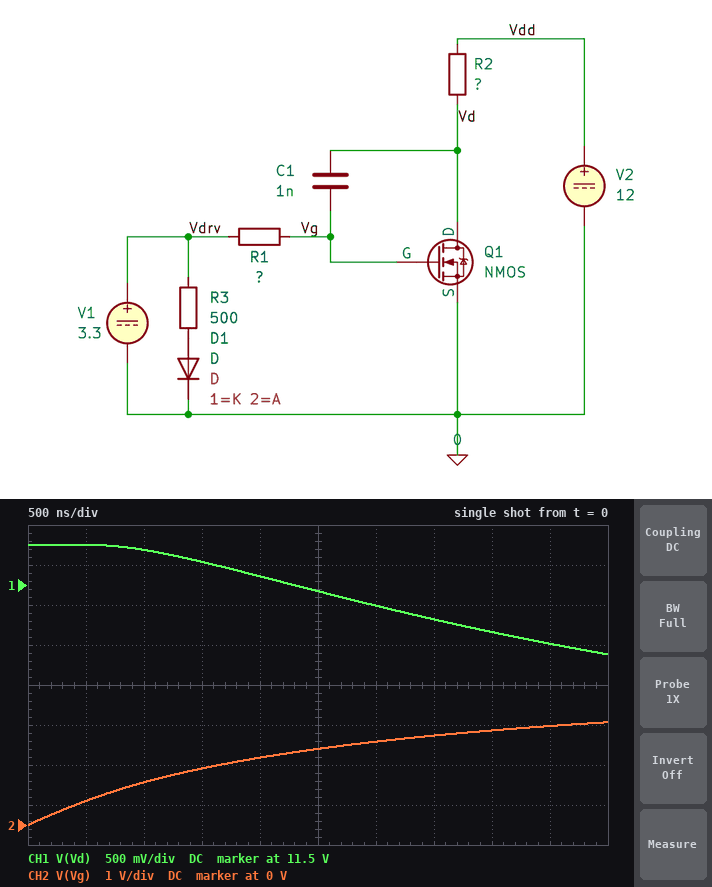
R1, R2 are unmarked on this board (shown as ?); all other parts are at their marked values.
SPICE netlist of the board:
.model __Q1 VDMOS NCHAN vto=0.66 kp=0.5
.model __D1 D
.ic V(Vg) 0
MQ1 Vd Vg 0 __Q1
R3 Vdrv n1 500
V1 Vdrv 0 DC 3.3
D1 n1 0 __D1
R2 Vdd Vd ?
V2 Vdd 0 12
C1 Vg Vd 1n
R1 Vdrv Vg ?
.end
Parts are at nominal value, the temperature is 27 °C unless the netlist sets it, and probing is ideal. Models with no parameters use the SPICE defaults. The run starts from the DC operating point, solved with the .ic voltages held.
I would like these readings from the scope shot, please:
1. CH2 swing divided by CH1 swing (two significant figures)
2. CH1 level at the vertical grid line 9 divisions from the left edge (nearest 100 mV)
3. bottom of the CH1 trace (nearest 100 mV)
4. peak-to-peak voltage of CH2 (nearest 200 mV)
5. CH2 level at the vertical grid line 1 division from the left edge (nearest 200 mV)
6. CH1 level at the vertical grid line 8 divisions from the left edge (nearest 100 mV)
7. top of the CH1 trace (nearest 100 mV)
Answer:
1.9
10.8 V
10.6 V
2.6 V
600 mV
10.9 V
12.0 V
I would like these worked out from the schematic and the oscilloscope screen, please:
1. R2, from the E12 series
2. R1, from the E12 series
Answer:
1.5 Ω
1 kΩ
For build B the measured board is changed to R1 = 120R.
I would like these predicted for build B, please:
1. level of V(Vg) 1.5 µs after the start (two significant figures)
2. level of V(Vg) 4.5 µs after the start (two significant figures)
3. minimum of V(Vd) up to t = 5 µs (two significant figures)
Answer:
3.2 V
3.3 V
9.4 V
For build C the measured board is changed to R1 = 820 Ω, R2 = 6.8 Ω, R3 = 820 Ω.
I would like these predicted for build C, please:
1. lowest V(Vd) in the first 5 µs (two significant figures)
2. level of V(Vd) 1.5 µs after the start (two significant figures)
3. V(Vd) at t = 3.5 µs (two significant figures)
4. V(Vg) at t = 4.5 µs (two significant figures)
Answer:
7.7 V
11 V
9.0 V
2.2 V
